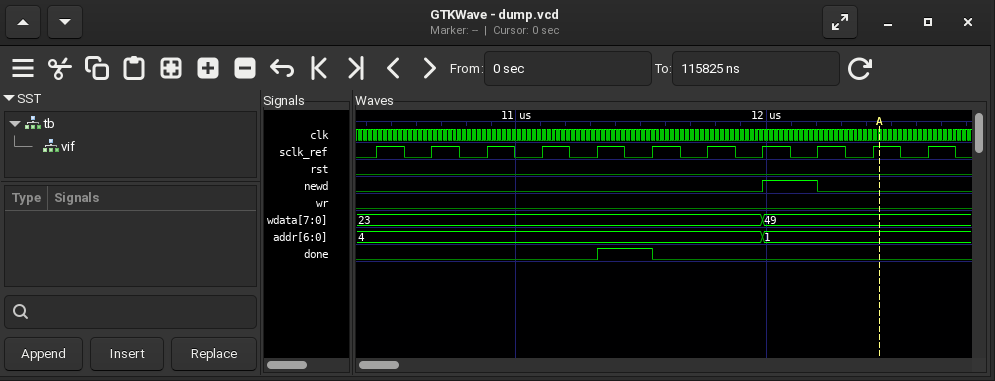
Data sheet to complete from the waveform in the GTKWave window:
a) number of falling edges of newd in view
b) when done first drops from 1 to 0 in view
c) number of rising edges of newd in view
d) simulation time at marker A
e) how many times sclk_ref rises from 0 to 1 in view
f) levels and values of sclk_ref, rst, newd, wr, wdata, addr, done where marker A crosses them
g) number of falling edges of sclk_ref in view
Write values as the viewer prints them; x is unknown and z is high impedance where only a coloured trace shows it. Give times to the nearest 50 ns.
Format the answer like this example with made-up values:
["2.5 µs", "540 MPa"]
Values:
["1", "11550 ns", "1", "12450 ns", "11", "sclk_ref=1, rst=0, newd=0, wr=0, wdata=49, addr=1, done=0", "11"]
